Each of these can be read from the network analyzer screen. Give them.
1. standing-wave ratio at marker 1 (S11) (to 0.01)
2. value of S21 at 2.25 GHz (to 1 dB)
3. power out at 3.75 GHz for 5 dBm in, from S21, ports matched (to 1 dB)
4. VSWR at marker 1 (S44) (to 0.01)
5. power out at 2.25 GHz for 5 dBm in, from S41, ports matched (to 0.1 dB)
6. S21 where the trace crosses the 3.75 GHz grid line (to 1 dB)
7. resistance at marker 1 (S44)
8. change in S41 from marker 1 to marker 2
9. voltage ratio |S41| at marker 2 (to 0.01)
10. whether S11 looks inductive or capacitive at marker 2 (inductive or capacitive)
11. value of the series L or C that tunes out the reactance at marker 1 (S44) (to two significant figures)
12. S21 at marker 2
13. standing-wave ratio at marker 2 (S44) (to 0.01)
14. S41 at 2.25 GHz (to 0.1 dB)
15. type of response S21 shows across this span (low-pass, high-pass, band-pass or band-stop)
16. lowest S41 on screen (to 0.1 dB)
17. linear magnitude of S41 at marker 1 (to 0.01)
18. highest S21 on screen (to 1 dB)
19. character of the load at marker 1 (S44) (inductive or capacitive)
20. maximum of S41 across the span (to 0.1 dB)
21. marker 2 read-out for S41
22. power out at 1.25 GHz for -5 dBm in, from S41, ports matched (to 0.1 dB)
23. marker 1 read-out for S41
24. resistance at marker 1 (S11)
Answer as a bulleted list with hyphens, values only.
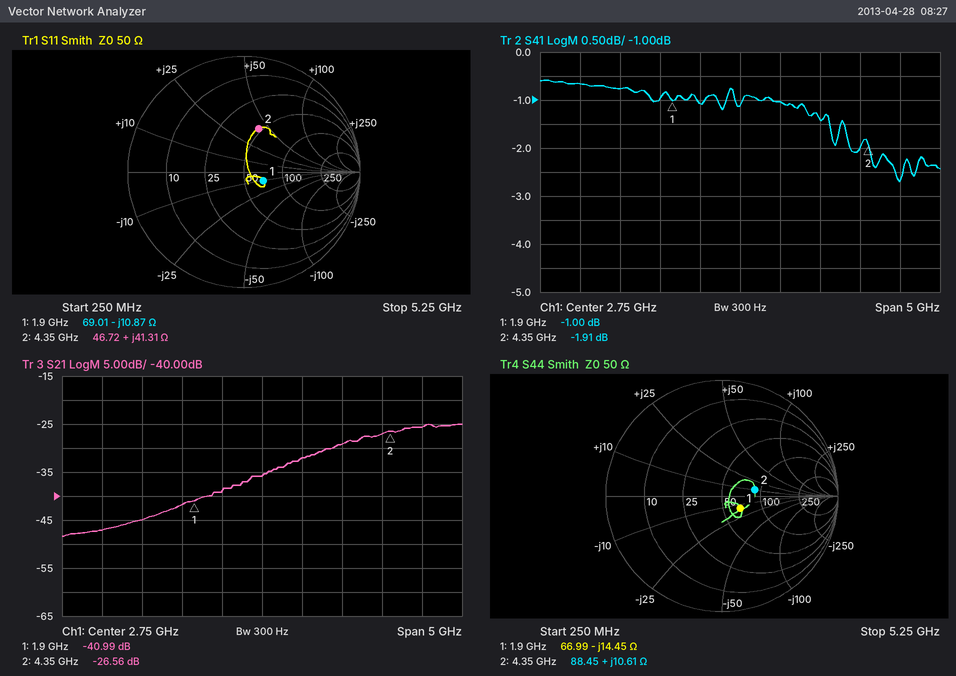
- 1.45
- -39 dB
- -24 dBm
- 1.47
- 3.9 dBm
- -29 dB
- 66.99 Ω
- -0.91 dB
- 0.80
- inductive
- 1.2 nH
- -26.56 dB
- 1.81
- -1.1 dB
- high-pass
- -2.7 dB
- 0.89
- -25 dB
- capacitive
- -0.6 dB
- -1.91 dB
- -5.8 dBm
- -1.00 dB
- 69.01 Ω
